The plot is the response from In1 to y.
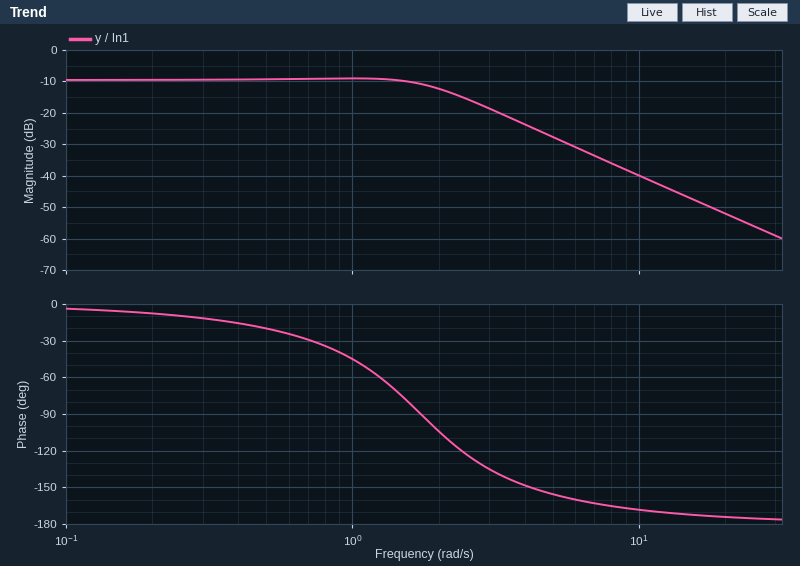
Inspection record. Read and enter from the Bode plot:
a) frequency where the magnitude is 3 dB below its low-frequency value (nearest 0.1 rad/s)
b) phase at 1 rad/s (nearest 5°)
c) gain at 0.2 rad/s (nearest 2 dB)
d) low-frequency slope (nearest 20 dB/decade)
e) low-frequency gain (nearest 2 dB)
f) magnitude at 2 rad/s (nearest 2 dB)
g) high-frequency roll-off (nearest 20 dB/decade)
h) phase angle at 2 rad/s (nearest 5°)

2.0 rad/s
-45°
-10 dB
0 dB/decade
-10 dB
-12 dB
-40 dB/decade
-105°
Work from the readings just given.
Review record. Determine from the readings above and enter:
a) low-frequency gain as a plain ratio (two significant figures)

0.32
